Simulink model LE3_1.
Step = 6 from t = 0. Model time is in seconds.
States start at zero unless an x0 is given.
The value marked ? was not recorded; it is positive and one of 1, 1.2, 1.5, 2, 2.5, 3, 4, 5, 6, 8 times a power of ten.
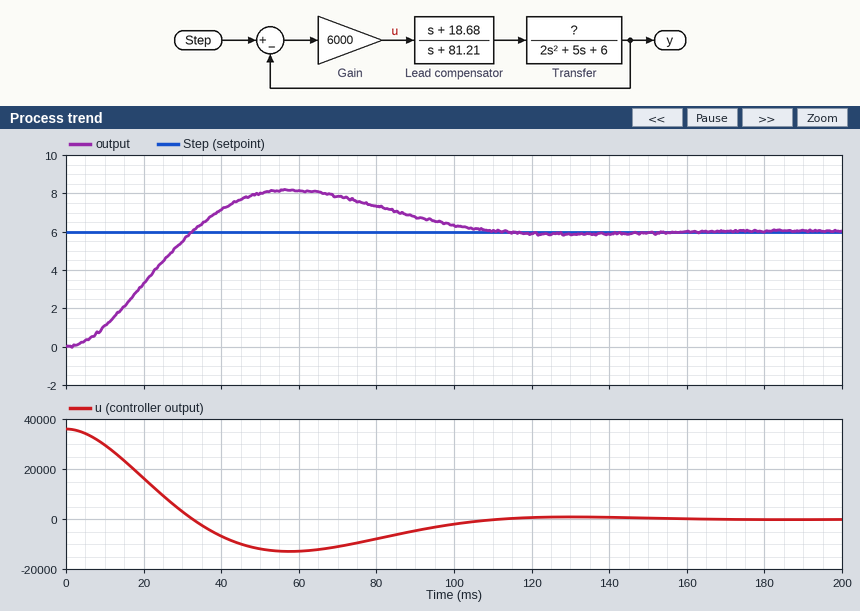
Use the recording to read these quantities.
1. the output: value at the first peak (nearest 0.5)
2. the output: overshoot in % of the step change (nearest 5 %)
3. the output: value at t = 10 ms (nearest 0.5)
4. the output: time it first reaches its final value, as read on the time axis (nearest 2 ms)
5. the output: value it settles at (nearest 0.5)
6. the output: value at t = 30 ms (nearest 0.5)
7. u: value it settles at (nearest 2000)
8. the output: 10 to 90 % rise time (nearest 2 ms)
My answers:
8.0
35 %
1.0
32 ms
6.0
5.5
0
22 ms
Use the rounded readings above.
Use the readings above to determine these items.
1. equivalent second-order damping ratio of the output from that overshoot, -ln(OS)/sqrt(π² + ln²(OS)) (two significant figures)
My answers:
0.32
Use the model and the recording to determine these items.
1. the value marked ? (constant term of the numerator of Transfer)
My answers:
1.5
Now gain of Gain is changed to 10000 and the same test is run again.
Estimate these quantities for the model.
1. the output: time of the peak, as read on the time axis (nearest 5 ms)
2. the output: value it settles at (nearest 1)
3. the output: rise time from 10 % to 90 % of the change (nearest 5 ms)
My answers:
40 ms
6
15 ms
